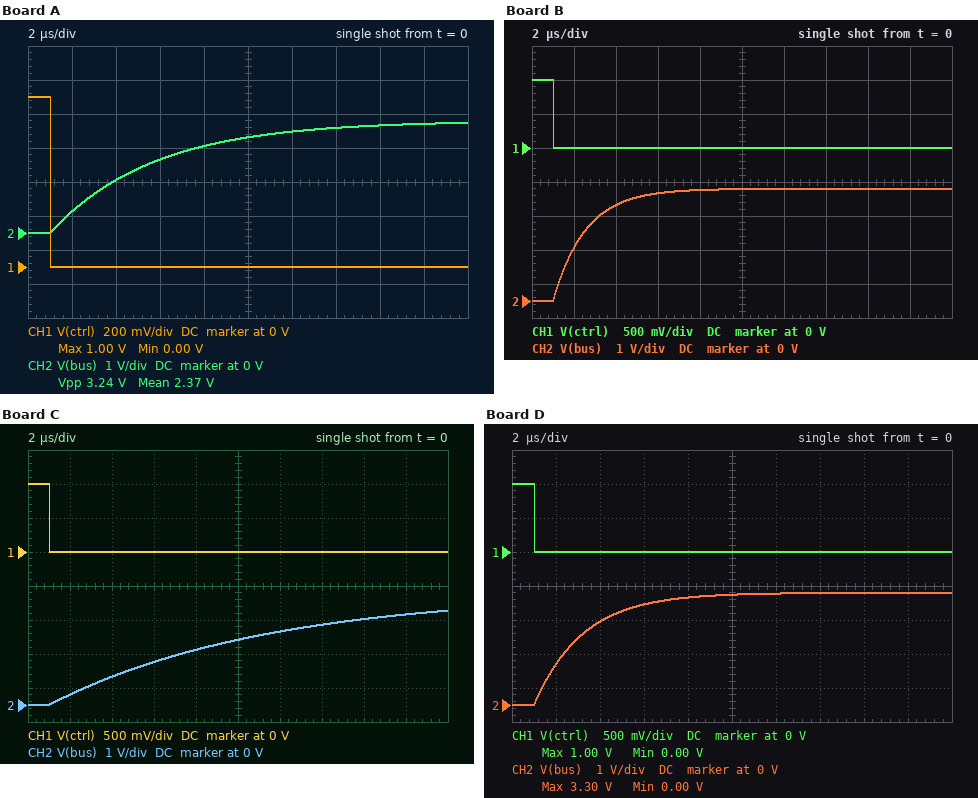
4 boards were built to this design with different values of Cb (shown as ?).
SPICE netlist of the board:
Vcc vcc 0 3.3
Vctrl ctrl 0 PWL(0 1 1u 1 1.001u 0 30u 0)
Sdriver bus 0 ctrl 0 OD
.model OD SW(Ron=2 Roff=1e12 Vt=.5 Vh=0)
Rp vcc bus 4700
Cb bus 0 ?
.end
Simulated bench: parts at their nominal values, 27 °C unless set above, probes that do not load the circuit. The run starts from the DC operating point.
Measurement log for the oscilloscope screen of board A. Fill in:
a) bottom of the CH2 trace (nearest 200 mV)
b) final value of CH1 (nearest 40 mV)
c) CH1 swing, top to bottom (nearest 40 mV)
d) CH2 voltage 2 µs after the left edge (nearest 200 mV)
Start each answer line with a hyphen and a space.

- 0 V
- 0 V
- 1.00 V
- 600 mV
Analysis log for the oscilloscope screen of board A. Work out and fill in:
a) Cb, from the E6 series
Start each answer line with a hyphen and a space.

- 1 nF
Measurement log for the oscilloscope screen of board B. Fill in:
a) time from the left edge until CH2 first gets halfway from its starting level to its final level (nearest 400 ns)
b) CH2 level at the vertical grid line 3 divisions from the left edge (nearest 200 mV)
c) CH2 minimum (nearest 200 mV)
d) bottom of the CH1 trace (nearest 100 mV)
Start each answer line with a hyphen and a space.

- 2.0 µs
- 3.2 V
- 0 V
- 0 V
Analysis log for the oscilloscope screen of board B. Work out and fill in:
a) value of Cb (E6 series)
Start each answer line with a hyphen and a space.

- 330 pF
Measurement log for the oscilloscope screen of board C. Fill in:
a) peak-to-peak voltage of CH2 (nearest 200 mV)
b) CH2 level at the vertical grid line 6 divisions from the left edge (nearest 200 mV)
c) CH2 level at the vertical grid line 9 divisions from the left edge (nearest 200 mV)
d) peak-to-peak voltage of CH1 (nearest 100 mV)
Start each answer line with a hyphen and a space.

- 2.8 V
- 2.2 V
- 2.6 V
- 1.0 V
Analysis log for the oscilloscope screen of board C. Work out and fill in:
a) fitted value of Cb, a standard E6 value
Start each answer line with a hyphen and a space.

- 2.2 nF
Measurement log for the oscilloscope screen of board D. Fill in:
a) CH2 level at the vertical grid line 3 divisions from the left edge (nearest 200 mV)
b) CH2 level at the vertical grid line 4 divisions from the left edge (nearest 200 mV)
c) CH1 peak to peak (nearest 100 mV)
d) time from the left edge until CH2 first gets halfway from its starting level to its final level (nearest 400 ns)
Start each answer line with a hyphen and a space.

- 3.0 V
- 3.2 V
- 1.0 V
- 2.4 µs
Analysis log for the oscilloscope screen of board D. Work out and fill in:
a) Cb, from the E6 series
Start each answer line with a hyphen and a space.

- 470 pF
